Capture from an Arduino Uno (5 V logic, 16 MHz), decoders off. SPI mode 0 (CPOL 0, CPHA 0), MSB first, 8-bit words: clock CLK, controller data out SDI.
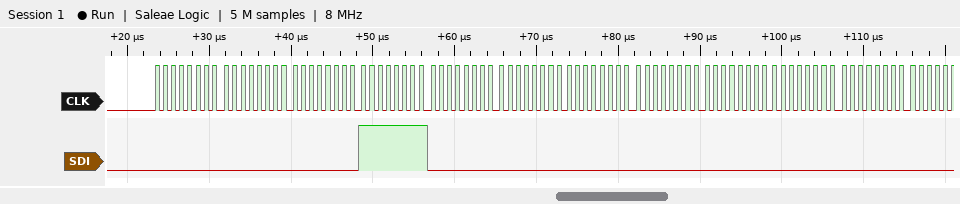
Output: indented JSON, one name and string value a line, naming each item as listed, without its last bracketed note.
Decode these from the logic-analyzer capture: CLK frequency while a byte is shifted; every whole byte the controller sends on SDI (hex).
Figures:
{
  "CLK frequency while a byte is shifted": "1 MHz",
  "every whole byte the controller sends on SDI": "00 00 00 FF 00 00 00 00 00 00 00"
}
